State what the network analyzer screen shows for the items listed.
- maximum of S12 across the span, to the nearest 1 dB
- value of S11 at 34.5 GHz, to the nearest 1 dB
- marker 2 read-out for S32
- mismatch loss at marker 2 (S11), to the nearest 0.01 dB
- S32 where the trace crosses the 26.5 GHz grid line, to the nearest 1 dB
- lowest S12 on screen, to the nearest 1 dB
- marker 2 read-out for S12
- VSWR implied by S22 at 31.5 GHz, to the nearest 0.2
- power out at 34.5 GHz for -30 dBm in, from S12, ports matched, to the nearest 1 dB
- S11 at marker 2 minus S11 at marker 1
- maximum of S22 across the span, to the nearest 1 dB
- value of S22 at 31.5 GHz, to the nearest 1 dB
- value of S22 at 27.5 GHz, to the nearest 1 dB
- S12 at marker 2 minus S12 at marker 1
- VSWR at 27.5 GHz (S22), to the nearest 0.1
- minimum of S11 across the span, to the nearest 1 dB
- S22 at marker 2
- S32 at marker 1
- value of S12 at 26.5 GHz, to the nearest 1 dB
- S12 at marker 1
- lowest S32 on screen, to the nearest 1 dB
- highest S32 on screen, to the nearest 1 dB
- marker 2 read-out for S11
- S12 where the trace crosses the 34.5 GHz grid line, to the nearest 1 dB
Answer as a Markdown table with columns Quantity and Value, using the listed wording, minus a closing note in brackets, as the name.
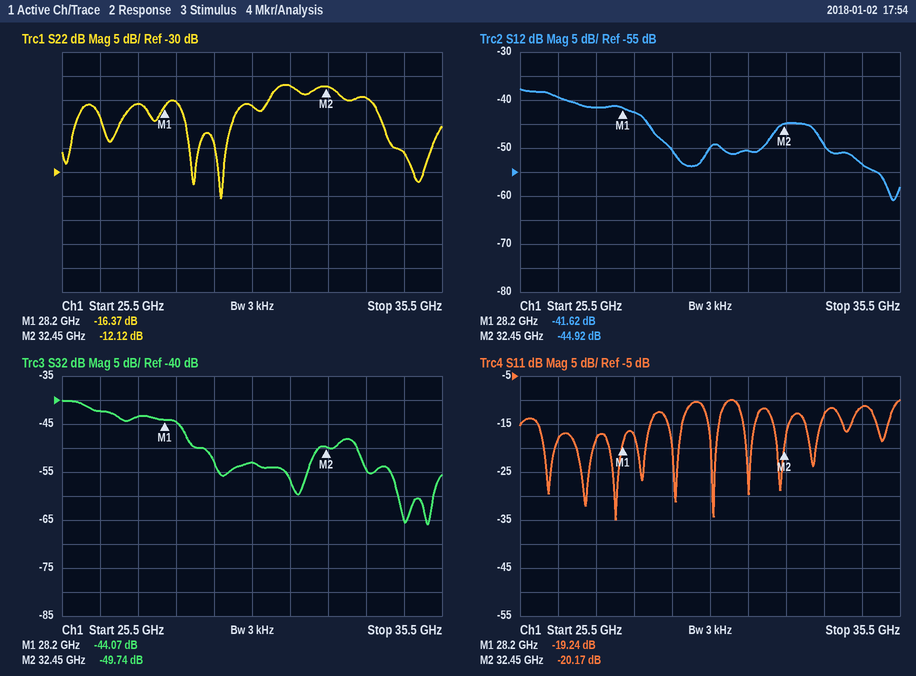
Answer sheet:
| Quantity | Value |
|---|---|
| maximum of S12 across the span, to the nearest 1 dB | -38 dB |
| value of S11 at 34.5 GHz, to the nearest 1 dB | -11 dB |
| marker 2 read-out for S32 | -49.74 dB |
| mismatch loss at marker 2 (S11), to the nearest 0.01 dB | 0.04 dB |
| S32 where the trace crosses the 26.5 GHz grid line, to the nearest 1 dB | -42 dB |
| lowest S12 on screen, to the nearest 1 dB | -61 dB |
| marker 2 read-out for S12 | -44.92 dB |
| VSWR implied by S22 at 31.5 GHz, to the nearest 0.2 | 1.6 |
| power out at 34.5 GHz for -30 dBm in, from S12, ports matched, to the nearest 1 dB | -83 dBm |
| S11 at marker 2 minus S11 at marker 1 | -0.93 dB |
| maximum of S22 across the span, to the nearest 1 dB | -12 dB |
| value of S22 at 31.5 GHz, to the nearest 1 dB | -12 dB |
| value of S22 at 27.5 GHz, to the nearest 1 dB | -16 dB |
| S12 at marker 2 minus S12 at marker 1 | -3.30 dB |
| VSWR at 27.5 GHz (S22), to the nearest 0.1 | 1.4 |
| minimum of S11 across the span, to the nearest 1 dB | -35 dB |
| S22 at marker 2 | -12.12 dB |
| S32 at marker 1 | -44.07 dB |
| value of S12 at 26.5 GHz, to the nearest 1 dB | -39 dB |
| S12 at marker 1 | -41.62 dB |
| lowest S32 on screen, to the nearest 1 dB | -66 dB |
| highest S32 on screen, to the nearest 1 dB | -40 dB |
| marker 2 read-out for S11 | -20.17 dB |
| S12 where the trace crosses the 34.5 GHz grid line, to the nearest 1 dB | -53 dB |
